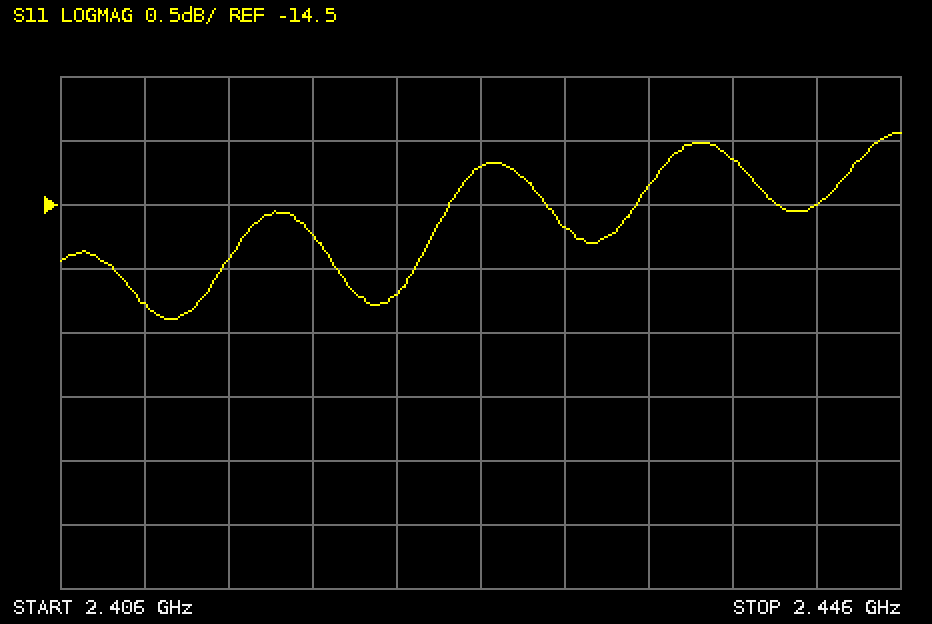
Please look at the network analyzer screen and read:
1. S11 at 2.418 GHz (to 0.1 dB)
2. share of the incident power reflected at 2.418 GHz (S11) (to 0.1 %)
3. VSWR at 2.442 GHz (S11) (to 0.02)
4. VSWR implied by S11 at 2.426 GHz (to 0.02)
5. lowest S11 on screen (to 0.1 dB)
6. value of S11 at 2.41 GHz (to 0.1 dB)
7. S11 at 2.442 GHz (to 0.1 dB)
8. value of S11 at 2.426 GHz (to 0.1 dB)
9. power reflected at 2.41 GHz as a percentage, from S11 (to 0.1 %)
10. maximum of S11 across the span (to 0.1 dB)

-14.7 dB
3.4 %
1.46
1.48
-15.4 dB
-15.3 dB
-14.5 dB
-14.2 dB
3.0 %
-13.9 dB
